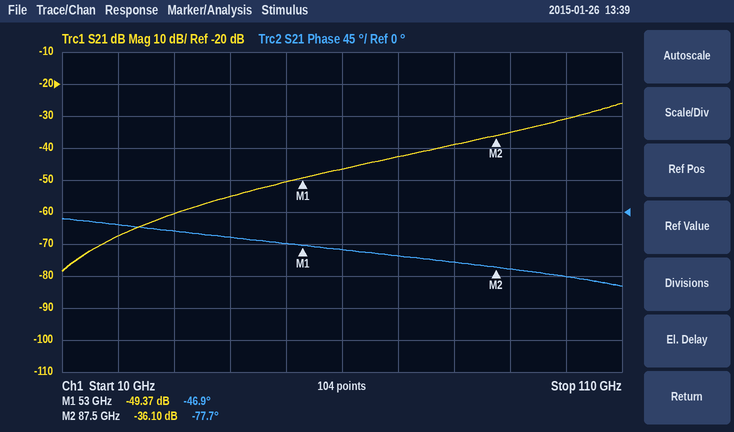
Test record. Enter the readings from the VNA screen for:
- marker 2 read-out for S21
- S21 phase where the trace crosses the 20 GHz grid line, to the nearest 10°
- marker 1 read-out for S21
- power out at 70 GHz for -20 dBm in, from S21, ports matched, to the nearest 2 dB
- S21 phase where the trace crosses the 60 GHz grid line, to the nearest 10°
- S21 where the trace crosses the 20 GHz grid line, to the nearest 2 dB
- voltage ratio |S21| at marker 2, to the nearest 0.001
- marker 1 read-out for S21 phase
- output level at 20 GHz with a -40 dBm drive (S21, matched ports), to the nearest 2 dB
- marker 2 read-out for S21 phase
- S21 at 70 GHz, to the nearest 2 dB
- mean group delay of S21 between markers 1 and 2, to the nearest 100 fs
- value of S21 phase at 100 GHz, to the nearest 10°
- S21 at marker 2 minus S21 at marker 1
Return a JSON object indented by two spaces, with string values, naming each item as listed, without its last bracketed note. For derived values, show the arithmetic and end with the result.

{
  "marker 2 read-out for S21": "-36.10 dB",
  "S21 phase where the trace crosses the 20 GHz grid line, to the nearest 10°": "-20°",
  "marker 1 read-out for S21": "-49.37 dB",
  "power out at 70 GHz for -20 dBm in, from S21, ports matched, to the nearest 2 dB": "-20 dBm + (-42 dB) = -62 dBm",
  "S21 phase where the trace crosses the 60 GHz grid line, to the nearest 10°": "-50°",
  "S21 where the trace crosses the 20 GHz grid line, to the nearest 2 dB": "-68 dB",
  "voltage ratio |S21| at marker 2, to the nearest 0.001": "10^(-36.1/20) ≈ 0.016",
  "marker 1 read-out for S21 phase": "-46.9°",
  "output level at 20 GHz with a -40 dBm drive (S21, matched ports), to the nearest 2 dB": "-40 dBm + (-68 dB) = -108 dBm",
  "marker 2 read-out for S21 phase": "-77.7°",
  "S21 at 70 GHz, to the nearest 2 dB": "-42 dB",
  "mean group delay of S21 between markers 1 and 2, to the nearest 100 fs": "−(-77.7° − (-46.9°))/(360° × 34.5 GHz) ≈ 2.5 ps",
  "value of S21 phase at 100 GHz, to the nearest 10°": "-90°",
  "S21 at marker 2 minus S21 at marker 1": "-36.1 − (-49.37) = 13.27 dB"
}
